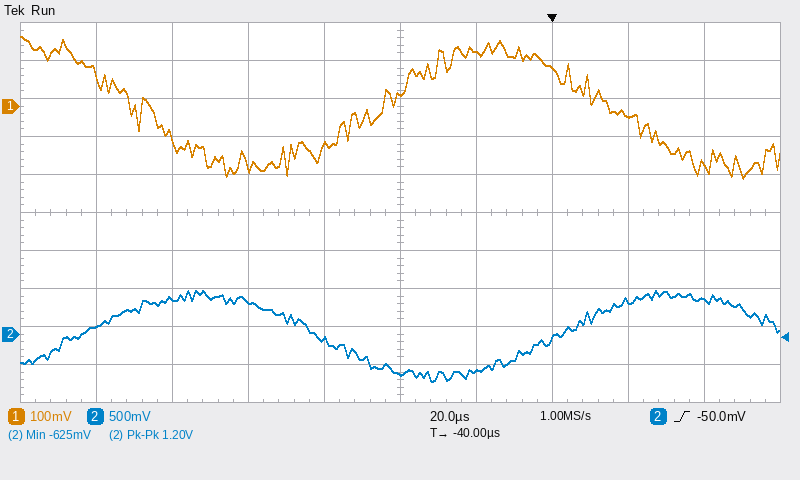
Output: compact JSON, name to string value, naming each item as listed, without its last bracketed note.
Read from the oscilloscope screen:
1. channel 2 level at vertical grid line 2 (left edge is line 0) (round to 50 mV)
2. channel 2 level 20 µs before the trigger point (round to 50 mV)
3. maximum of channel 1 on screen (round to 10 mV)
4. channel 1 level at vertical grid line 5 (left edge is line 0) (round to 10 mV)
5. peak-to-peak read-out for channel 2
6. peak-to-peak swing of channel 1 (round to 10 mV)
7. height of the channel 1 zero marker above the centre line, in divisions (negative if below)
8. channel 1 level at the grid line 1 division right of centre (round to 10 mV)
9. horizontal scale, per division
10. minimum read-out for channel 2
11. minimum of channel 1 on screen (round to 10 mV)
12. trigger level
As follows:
{"channel 2 level at vertical grid line 2 (left edge is line 0)": "450 mV", "channel 2 level 20 µs before the trigger point": "-500 mV", "maximum of channel 1 on screen": "180 mV", "channel 1 level at vertical grid line 5 (left edge is line 0)": "30 mV", "peak-to-peak read-out for channel 2": "1.20 V", "peak-to-peak swing of channel 1": "370 mV", "height of the channel 1 zero marker above the centre line, in divisions": "+2.8 div", "channel 1 level at the grid line 1 division right of centre": "140 mV", "horizontal scale, per division": "20 µs", "minimum read-out for channel 2": "-625 mV", "minimum of channel 1 on screen": "-190 mV", "trigger level": "-50.0 mV"}
